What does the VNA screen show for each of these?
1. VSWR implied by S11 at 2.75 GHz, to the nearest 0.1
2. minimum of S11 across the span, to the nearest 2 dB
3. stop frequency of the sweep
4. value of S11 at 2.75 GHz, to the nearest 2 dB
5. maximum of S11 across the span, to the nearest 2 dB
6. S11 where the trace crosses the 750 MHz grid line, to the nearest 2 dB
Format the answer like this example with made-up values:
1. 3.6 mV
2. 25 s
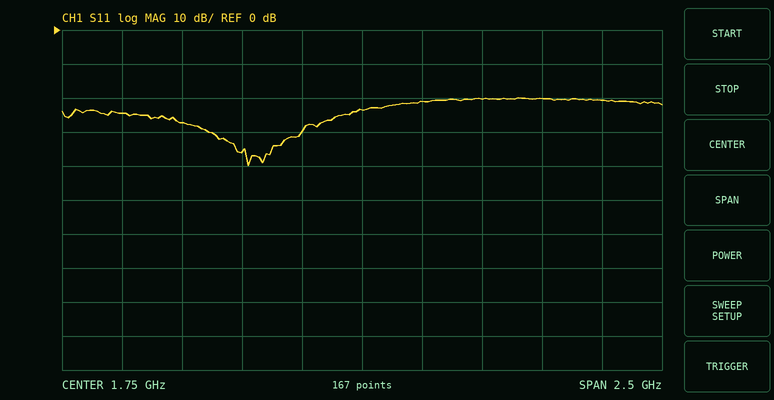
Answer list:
1. 1.2
2. -40 dB
3. 3 GHz
4. -20 dB
5. -20 dB
6. -24 dB
